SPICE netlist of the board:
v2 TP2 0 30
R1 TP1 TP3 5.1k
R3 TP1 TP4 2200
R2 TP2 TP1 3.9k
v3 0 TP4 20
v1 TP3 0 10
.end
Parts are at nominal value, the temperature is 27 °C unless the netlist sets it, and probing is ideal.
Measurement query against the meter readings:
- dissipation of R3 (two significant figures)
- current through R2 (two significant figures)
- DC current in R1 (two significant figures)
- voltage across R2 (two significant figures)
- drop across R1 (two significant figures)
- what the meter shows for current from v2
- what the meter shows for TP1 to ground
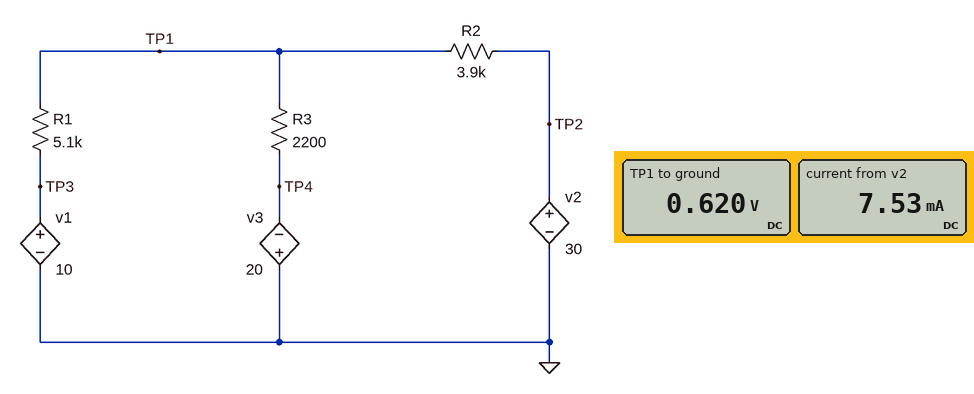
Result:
190 mW
7.5 mA
1.8 mA
29 V
9.4 V
7.53 mA
0.620 V
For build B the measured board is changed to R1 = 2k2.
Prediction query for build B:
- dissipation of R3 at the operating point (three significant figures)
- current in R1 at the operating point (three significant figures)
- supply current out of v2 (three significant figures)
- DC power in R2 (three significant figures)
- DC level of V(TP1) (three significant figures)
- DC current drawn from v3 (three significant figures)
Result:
234 mW
3.32 mA
7.00 mA
191 mW
2.70 V
10.3 mA
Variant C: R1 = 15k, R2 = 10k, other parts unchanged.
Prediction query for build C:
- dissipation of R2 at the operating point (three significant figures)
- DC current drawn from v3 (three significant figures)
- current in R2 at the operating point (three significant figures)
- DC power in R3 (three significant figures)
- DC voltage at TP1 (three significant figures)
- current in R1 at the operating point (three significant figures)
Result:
150 mW
5.12 mA
3.87 mA
57.7 mW
-8.73 V
1.25 mA
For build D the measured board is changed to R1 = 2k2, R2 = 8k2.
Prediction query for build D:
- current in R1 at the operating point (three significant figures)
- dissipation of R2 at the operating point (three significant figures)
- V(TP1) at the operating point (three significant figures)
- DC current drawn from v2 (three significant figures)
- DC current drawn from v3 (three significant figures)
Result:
4.94 mA
116 mW
-860 mV
3.76 mA
8.70 mA
